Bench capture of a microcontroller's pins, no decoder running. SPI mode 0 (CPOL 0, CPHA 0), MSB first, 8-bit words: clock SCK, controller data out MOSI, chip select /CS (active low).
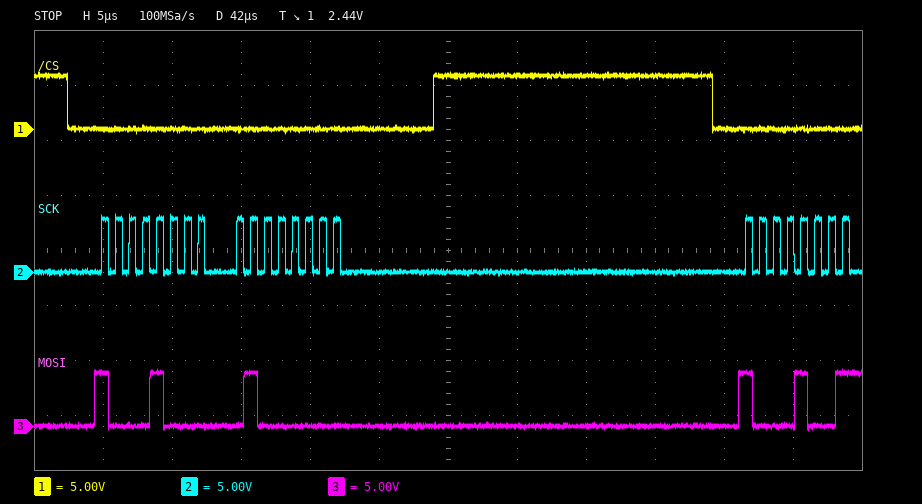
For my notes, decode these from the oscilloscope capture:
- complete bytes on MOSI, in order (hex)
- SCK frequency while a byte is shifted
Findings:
88 40 89
1 MHz
